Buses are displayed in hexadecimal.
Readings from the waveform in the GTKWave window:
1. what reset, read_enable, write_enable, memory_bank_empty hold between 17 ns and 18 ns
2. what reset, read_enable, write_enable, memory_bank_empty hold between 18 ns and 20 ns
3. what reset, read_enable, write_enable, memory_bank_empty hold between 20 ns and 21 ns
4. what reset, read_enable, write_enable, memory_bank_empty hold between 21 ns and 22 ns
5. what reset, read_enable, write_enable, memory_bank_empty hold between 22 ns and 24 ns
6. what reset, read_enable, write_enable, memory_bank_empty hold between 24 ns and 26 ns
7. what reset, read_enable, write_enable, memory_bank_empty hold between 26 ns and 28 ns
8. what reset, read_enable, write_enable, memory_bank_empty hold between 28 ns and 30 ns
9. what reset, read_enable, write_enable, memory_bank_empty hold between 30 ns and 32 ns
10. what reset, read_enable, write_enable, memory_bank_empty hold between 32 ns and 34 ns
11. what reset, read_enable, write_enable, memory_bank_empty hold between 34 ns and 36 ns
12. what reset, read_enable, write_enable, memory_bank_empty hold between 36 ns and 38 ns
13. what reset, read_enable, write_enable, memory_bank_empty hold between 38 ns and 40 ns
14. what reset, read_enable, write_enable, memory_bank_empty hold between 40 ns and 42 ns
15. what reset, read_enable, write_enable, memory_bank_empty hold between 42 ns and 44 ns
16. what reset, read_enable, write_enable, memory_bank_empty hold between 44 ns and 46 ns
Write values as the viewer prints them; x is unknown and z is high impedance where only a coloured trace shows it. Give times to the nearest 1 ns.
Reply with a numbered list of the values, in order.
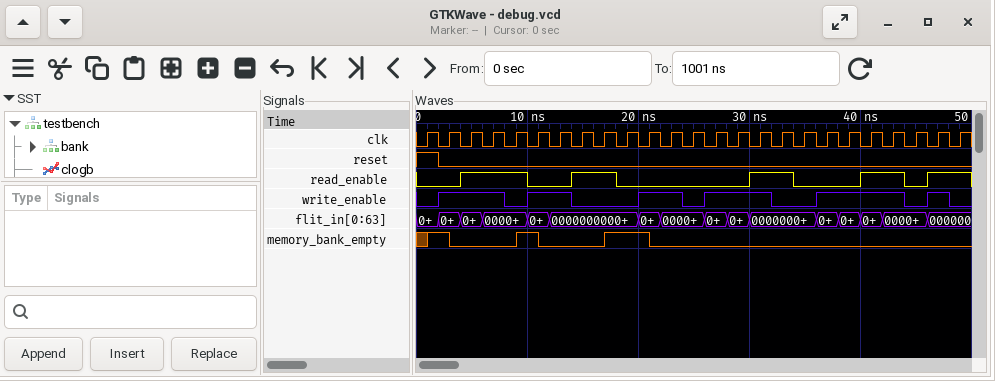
1. reset=0, read_enable=1, write_enable=0, memory_bank_empty=1
2. reset=0, read_enable=0, write_enable=0, memory_bank_empty=1
3. reset=0, read_enable=0, write_enable=1, memory_bank_empty=1
4. reset=0, read_enable=0, write_enable=1, memory_bank_empty=0
5. reset=0, read_enable=0, write_enable=1, memory_bank_empty=0
6. reset=0, read_enable=0, write_enable=0, memory_bank_empty=0
7. reset=0, read_enable=0, write_enable=1, memory_bank_empty=0
8. reset=0, read_enable=0, write_enable=1, memory_bank_empty=0
9. reset=0, read_enable=1, write_enable=1, memory_bank_empty=0
10. reset=0, read_enable=1, write_enable=0, memory_bank_empty=0
11. reset=0, read_enable=0, write_enable=0, memory_bank_empty=0
12. reset=0, read_enable=0, write_enable=1, memory_bank_empty=0
13. reset=0, read_enable=0, write_enable=1, memory_bank_empty=0
14. reset=0, read_enable=1, write_enable=1, memory_bank_empty=0
15. reset=0, read_enable=1, write_enable=1, memory_bank_empty=0
16. reset=0, read_enable=0, write_enable=0, memory_bank_empty=0
